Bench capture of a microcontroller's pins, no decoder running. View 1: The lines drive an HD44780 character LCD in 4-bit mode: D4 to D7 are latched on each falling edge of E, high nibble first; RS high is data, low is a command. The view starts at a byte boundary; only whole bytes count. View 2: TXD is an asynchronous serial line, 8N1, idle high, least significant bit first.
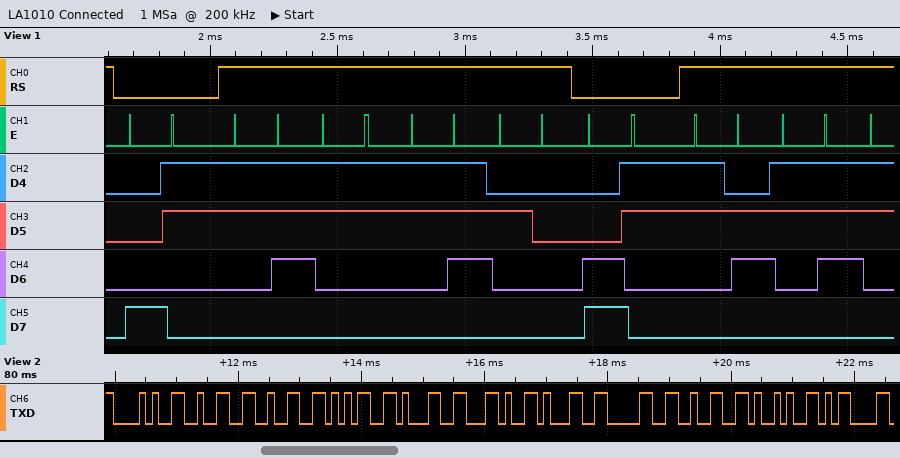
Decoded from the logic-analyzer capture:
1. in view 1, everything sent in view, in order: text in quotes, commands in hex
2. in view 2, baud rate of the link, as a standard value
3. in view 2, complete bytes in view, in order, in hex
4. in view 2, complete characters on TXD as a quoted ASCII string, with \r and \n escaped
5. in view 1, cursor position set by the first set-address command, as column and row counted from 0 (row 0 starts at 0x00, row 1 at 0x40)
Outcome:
0x83 "737 " 0xC3 "67"
9600 baud
28 32 32 35 31 2C 31 30 32 29 0D
"(2251,102)\r"
column 3, row 0
